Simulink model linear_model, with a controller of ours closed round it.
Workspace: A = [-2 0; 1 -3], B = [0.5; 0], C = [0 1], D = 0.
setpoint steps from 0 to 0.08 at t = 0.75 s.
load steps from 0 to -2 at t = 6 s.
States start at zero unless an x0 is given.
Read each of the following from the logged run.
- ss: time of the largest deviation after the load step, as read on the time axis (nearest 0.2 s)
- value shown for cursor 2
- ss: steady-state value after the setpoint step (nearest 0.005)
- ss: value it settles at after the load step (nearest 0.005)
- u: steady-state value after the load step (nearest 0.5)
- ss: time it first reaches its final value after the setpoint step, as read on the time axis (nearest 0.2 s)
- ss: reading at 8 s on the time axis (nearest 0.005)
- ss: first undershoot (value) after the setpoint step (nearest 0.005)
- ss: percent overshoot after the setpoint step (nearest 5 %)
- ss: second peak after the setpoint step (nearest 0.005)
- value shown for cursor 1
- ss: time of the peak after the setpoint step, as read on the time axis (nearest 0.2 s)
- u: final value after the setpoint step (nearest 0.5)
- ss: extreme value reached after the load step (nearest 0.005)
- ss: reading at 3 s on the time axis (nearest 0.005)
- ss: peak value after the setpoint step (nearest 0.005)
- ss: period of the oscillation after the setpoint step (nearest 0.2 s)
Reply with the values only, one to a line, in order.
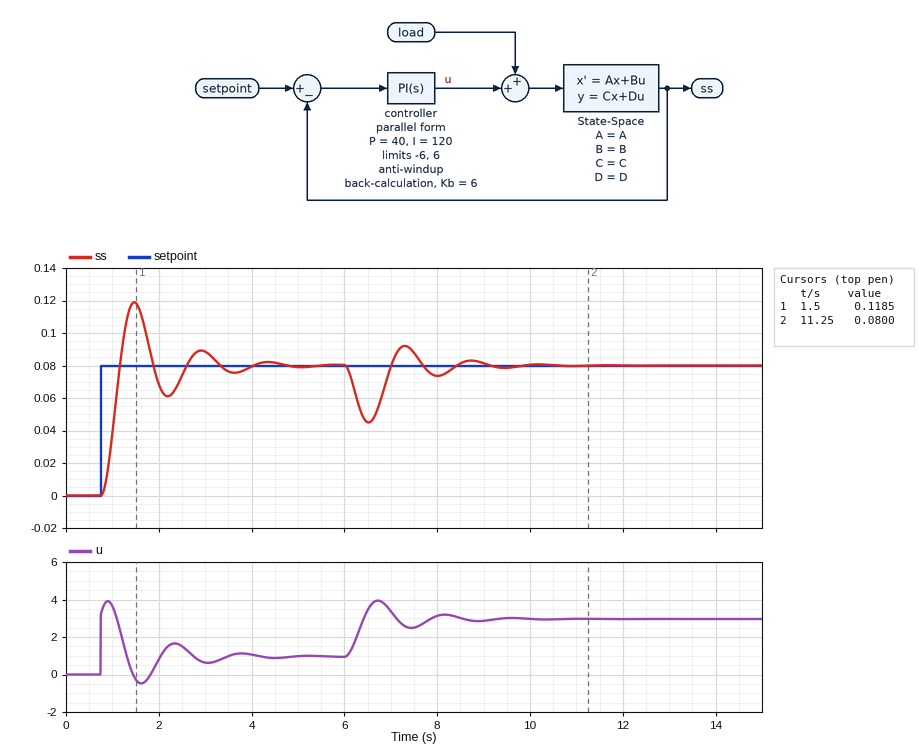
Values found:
6.6 s
0.0800
0.080
0.080
3.0
1.2 s
0.075
0.060
50 %
0.090
0.1185
1.4 s
1.0
0.045
0.090
0.120
1.4 s
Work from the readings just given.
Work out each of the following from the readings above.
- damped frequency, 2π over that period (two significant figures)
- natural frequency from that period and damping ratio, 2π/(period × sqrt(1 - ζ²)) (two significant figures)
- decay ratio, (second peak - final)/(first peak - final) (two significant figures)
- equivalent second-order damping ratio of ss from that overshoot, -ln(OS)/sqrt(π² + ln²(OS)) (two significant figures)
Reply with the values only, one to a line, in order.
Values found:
4.5 rad/s
4.6 rad/s
0.25
0.22
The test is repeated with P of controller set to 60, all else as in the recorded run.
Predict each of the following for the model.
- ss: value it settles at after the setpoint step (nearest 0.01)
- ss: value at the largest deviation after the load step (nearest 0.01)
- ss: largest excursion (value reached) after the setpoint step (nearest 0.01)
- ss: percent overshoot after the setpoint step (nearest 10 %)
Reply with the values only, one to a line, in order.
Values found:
0.08
0.05
0.11
40 %
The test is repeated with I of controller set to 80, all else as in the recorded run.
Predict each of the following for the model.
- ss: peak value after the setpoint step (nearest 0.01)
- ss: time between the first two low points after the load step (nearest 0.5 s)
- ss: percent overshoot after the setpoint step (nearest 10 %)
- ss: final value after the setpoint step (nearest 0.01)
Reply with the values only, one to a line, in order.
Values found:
0.11
1.5 s
30 %
0.08
